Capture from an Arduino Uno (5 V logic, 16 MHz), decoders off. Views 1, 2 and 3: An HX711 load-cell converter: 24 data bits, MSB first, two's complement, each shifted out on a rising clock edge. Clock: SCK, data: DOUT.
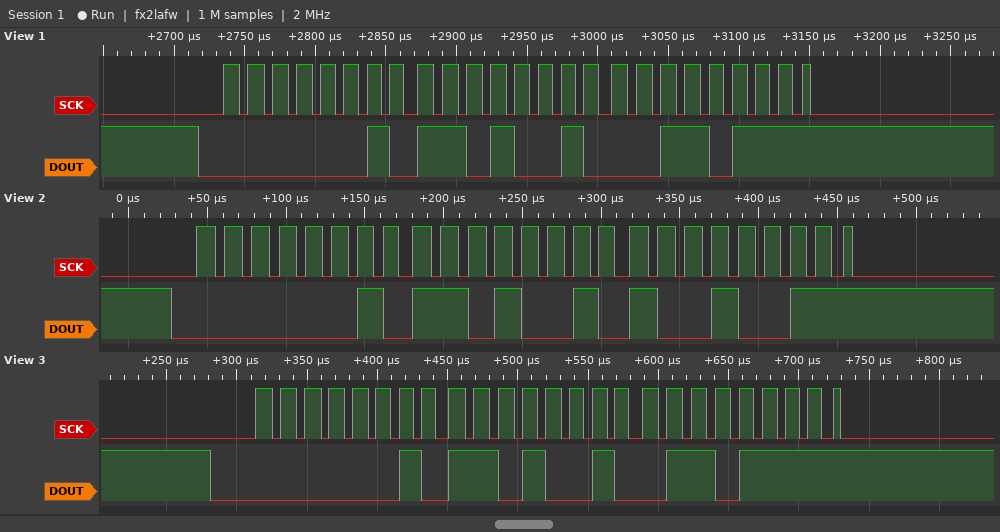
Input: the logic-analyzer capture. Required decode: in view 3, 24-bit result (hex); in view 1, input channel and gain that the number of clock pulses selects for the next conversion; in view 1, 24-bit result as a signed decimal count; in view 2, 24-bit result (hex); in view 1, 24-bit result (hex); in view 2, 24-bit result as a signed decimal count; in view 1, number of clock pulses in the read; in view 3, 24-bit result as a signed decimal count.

0x02D26F
channel A, gain 128
184887
0x02D293
0x02D237
184979
25
184943
